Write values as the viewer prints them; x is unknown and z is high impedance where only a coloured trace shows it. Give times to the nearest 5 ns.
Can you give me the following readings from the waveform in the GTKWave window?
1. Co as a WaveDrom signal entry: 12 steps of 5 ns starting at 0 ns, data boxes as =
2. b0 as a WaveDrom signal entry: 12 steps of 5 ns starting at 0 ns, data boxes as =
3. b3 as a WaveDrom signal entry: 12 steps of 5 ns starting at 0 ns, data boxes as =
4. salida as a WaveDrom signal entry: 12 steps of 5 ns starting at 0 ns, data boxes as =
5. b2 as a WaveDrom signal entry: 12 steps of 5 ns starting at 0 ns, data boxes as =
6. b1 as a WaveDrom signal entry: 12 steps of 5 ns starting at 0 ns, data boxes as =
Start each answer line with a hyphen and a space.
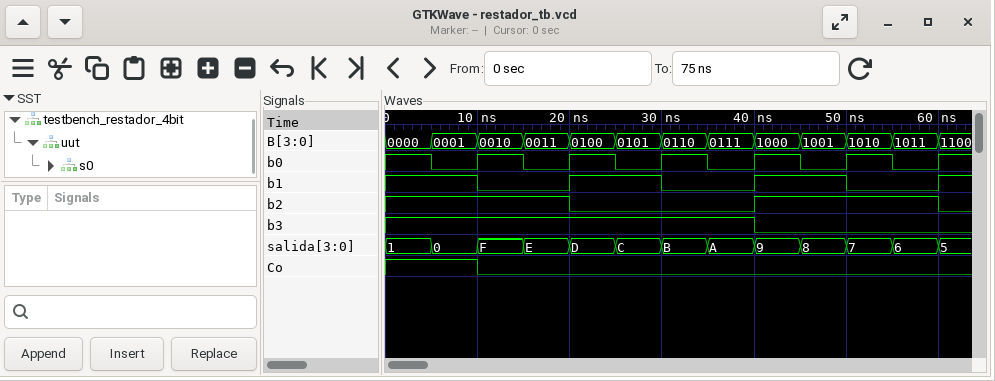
- {name: 'Co', wave: '1.0.........'}
- {name: 'b0', wave: '101010101010'}
- {name: 'b3', wave: '1.......0...'}
- {name: 'salida', wave: '============', data: '1 0 F E D C B A 9 8 7 6'}
- {name: 'b2', wave: '1...0...1...'}
- {name: 'b1', wave: '1.0.1.0.1.0.'}
